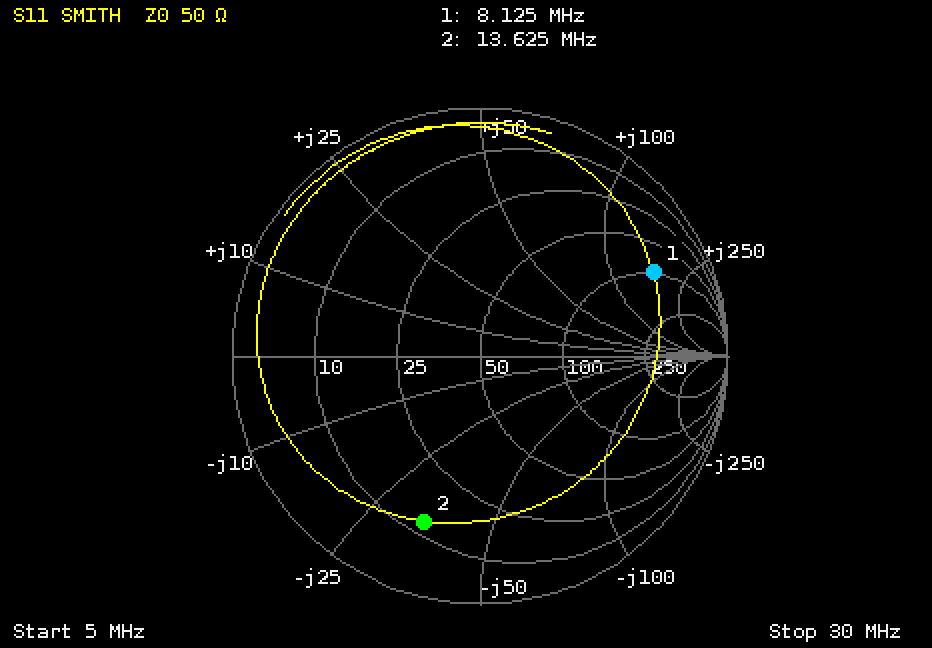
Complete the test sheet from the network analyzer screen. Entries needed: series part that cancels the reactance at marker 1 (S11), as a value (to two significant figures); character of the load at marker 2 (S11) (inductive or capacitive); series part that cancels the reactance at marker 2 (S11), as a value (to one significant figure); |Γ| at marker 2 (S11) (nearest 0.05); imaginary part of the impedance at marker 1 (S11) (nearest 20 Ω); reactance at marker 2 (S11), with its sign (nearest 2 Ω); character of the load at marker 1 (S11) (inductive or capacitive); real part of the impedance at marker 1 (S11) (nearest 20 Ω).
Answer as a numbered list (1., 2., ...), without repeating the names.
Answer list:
1. 120 pF
2. capacitive
3. 400 nH
4. 0.70
5. +160 Ω
6. -34 Ω
7. inductive
8. 100 Ω
